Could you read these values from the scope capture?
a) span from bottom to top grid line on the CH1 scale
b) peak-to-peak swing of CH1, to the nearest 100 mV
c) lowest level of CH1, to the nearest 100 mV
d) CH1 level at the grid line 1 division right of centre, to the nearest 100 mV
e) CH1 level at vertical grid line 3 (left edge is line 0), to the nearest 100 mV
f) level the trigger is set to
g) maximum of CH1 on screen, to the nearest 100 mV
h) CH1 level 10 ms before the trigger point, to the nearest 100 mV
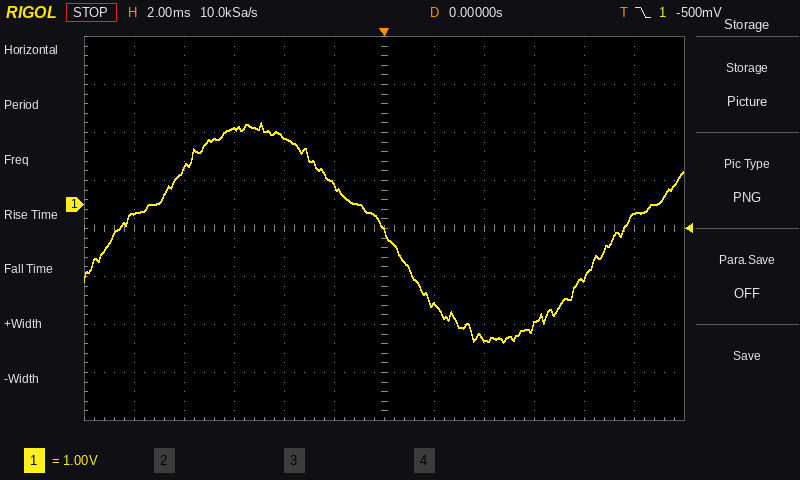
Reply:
8 V
4.6 V
-2.9 V
-2.1 V
1.6 V
-500 mV
1.7 V
-200 mV
